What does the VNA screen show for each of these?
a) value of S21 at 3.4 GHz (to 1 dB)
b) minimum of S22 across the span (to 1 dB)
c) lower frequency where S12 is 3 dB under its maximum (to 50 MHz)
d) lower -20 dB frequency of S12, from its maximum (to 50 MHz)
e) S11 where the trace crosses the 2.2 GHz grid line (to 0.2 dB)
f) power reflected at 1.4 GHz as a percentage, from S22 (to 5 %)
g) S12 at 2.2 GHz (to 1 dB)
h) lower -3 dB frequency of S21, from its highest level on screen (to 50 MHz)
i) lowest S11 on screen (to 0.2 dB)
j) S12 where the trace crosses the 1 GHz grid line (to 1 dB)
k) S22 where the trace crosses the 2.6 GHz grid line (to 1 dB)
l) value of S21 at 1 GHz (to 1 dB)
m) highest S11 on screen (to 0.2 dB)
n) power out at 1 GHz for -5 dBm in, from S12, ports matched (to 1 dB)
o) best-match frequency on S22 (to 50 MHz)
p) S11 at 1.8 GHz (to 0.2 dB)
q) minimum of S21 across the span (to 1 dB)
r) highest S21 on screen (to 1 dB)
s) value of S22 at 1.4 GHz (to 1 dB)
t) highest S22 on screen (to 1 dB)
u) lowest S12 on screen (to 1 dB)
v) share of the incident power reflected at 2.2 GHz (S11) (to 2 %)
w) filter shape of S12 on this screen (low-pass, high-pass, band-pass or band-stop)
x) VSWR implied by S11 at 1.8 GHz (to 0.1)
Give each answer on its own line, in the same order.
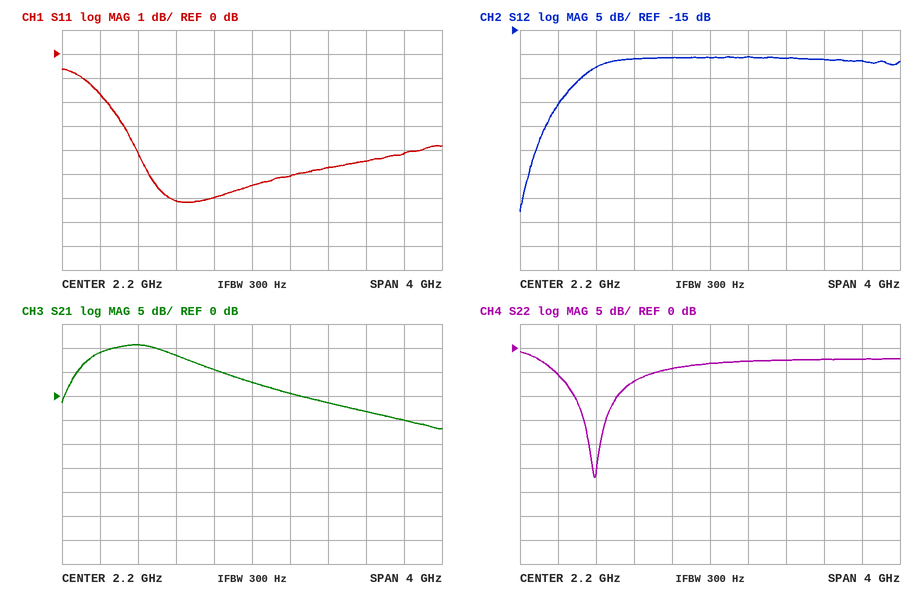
-3 dB
-27 dB
950 MHz
350 MHz
-5.4 dB
20 %
-21 dB
500 MHz
-6.2 dB
-23 dB
-3 dB
11 dB
-0.6 dB
-28 dBm
1.00 GHz
-6.0 dB
-7 dB
11 dB
-7 dB
-1 dB
-53 dB
28 %
high-pass
3.0
